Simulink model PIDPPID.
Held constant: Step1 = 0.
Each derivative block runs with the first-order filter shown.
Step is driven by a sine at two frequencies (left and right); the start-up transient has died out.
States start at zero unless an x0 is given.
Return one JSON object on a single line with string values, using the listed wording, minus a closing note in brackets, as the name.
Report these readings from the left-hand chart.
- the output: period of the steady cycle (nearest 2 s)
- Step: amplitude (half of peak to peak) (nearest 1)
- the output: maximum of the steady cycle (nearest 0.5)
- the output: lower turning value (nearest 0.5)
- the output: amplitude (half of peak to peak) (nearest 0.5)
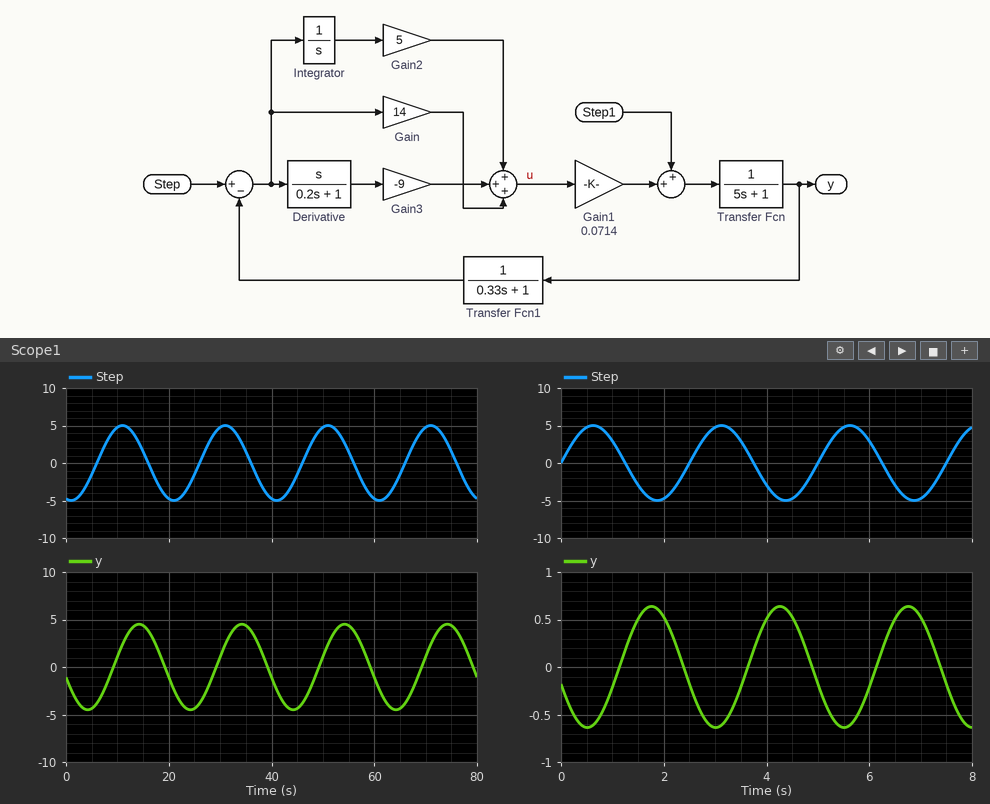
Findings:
{"the output: period of the steady cycle": "20 s", "Step: amplitude (half of peak to peak)": "5", "the output: maximum of the steady cycle": "4.5", "the output: lower turning value": "-4.5", "the output: amplitude (half of peak to peak)": "4.5"}
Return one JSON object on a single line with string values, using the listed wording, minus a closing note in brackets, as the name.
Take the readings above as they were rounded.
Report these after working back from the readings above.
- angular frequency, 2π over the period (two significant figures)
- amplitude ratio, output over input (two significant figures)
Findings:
{"angular frequency, 2π over the period": "0.31 rad/s", "amplitude ratio, output over input": "0.90"}
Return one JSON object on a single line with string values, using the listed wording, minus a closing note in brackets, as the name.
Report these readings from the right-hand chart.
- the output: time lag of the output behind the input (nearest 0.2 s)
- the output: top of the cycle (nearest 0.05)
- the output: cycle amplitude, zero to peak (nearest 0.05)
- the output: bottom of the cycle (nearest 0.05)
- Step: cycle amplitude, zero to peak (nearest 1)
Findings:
{"the output: time lag of the output behind the input": "1.2 s", "the output: top of the cycle": "0.65", "the output: cycle amplitude, zero to peak": "0.65", "the output: bottom of the cycle": "-0.65", "Step: cycle amplitude, zero to peak": "5"}
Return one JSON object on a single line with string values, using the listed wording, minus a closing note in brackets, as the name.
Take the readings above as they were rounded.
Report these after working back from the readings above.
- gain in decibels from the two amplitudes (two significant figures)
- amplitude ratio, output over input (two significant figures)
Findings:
{"gain in decibels from the two amplitudes": "-18 dB", "amplitude ratio, output over input": "0.13"}
